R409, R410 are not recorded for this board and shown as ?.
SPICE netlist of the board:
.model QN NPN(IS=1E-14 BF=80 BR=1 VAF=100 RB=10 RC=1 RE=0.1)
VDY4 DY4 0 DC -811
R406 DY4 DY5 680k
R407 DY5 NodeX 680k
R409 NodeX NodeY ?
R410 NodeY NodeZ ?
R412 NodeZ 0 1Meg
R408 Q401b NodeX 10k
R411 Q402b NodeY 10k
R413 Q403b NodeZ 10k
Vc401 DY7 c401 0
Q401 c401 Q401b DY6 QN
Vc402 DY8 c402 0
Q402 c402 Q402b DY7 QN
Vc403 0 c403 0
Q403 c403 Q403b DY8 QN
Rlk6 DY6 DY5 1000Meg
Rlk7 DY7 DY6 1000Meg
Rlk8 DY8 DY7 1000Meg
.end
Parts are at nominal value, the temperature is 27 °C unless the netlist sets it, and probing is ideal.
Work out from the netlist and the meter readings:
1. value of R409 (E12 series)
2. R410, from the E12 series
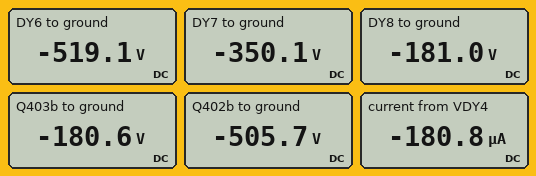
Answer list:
330 kΩ
1.8 MΩ
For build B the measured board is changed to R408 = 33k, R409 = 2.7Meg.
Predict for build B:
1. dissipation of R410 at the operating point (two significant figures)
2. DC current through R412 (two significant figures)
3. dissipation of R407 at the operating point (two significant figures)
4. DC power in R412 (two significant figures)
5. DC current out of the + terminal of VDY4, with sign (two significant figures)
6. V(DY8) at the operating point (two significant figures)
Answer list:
25 mW
120 µA
9.5 mW
14 mW
-120 µA
-120 V
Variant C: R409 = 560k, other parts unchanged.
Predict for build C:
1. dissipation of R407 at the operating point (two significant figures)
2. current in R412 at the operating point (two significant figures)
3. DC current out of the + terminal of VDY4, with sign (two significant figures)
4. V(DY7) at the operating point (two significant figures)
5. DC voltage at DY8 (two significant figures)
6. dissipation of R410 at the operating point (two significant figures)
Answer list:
20 mW
170 µA
-170 µA
-350 V
-170 V
53 mW
